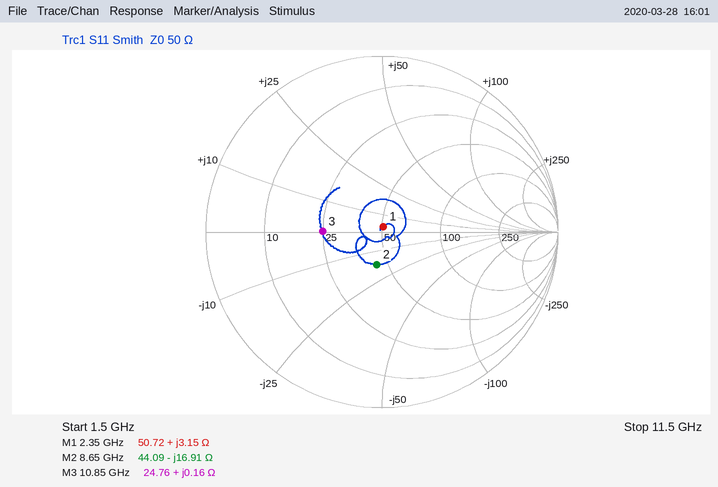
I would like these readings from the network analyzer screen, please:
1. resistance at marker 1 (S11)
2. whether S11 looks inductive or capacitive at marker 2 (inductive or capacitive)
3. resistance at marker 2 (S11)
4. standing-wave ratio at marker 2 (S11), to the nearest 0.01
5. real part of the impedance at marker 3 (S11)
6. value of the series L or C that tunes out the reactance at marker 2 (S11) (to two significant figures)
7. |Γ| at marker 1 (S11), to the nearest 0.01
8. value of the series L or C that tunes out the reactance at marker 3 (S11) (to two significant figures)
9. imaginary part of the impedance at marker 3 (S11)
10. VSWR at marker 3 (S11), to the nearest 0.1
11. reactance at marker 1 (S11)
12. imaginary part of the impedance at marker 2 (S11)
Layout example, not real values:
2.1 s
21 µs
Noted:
50.72 Ω
capacitive
44.09 Ω
1.46
24.76 Ω
310 pH
0.03
92 pF
+0.16 Ω
2.0
+3.15 Ω
-16.91 Ω
